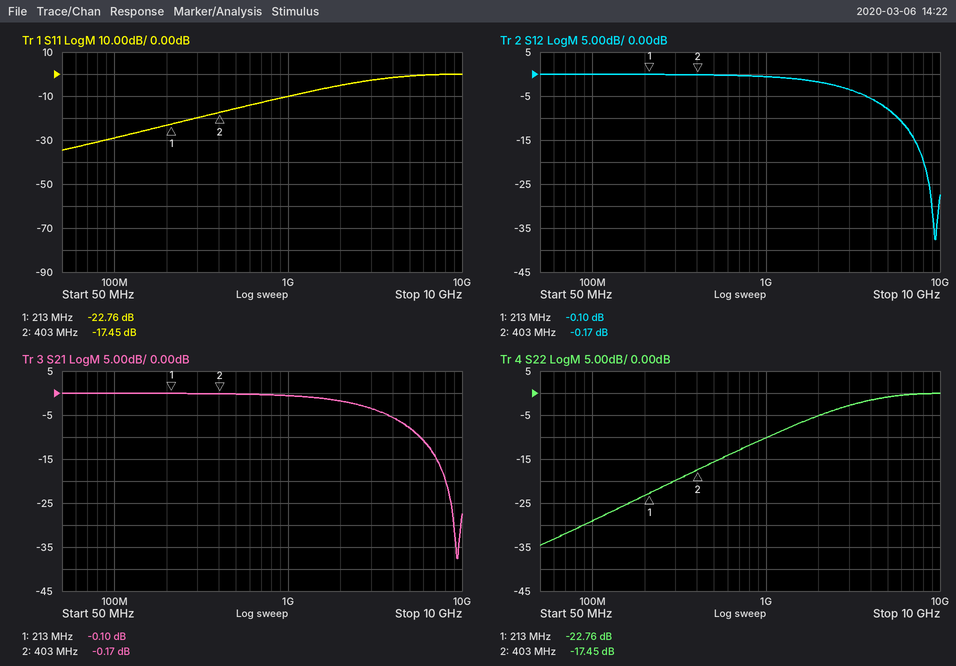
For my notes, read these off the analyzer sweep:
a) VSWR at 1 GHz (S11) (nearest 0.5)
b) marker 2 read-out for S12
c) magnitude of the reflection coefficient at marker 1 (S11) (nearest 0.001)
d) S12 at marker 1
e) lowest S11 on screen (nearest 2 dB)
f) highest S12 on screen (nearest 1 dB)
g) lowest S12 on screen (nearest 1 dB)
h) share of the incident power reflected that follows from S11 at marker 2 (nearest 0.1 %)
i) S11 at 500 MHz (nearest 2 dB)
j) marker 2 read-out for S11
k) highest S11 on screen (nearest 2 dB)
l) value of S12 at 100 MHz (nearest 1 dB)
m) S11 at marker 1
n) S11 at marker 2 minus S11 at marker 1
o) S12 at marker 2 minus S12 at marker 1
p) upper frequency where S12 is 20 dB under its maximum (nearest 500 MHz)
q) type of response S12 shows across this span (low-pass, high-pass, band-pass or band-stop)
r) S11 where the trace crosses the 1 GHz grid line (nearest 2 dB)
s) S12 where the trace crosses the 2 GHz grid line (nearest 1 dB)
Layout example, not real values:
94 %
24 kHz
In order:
2.0
-0.17 dB
0.073
-0.10 dB
-34 dB
0 dB
-38 dB
1.8 %
-16 dB
-17.45 dB
0 dB
0 dB
-22.76 dB
5.31 dB
-0.07 dB
8.0 GHz
low-pass
-10 dB
-2 dB
